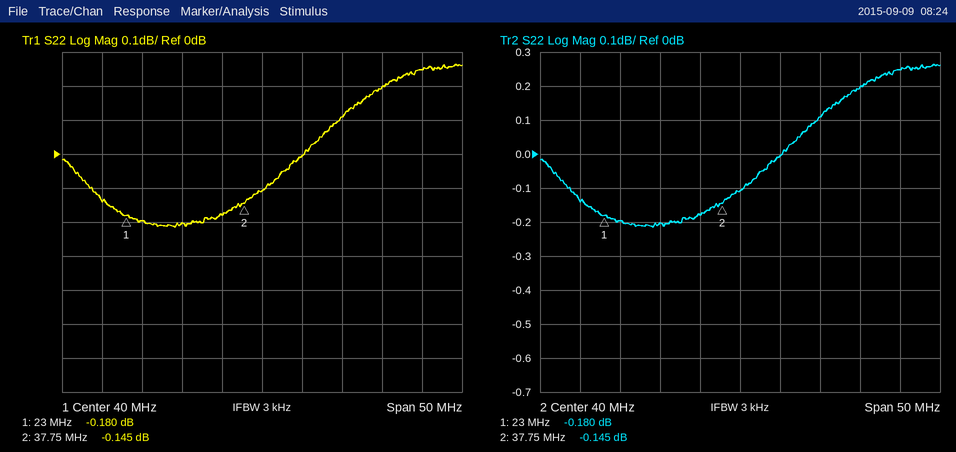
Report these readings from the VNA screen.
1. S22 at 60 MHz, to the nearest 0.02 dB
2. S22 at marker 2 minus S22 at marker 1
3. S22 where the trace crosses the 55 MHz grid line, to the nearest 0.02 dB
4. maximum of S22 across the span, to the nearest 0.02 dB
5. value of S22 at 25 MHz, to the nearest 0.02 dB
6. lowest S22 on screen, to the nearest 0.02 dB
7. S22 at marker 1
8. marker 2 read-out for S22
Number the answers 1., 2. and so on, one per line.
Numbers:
1. 0.24 dB
2. 0.035 dB
3. 0.20 dB
4. 0.26 dB
5. -0.20 dB
6. -0.22 dB
7. -0.180 dB
8. -0.145 dB
